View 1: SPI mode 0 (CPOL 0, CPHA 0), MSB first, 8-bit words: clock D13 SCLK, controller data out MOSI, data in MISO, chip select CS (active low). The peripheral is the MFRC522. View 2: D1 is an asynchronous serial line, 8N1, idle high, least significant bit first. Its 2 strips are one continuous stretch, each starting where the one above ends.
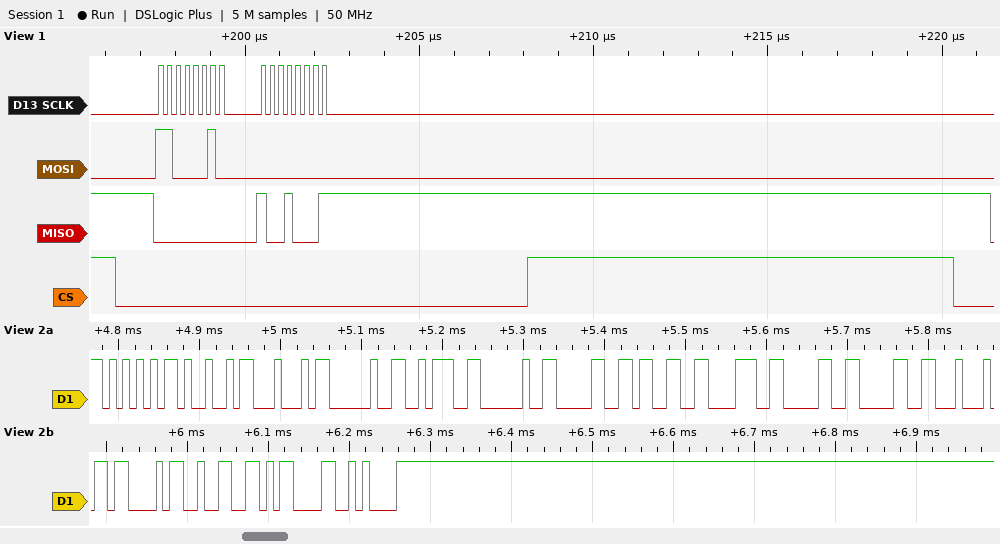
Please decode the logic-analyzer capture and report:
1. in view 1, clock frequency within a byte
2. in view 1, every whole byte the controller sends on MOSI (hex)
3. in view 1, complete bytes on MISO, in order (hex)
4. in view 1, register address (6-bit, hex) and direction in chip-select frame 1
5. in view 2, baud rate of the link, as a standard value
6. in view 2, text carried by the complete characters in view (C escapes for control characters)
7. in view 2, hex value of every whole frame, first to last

4 MHz
C2 00
00 91
0x21 read
115200 baud
"UID : 03800DC2\r\n"
0x55 0x49 0x44 0x20 0x3A 0x20 0x30 0x33 0x38 0x30 0x30 0x44 0x43 0x32 0x0D 0x0A
